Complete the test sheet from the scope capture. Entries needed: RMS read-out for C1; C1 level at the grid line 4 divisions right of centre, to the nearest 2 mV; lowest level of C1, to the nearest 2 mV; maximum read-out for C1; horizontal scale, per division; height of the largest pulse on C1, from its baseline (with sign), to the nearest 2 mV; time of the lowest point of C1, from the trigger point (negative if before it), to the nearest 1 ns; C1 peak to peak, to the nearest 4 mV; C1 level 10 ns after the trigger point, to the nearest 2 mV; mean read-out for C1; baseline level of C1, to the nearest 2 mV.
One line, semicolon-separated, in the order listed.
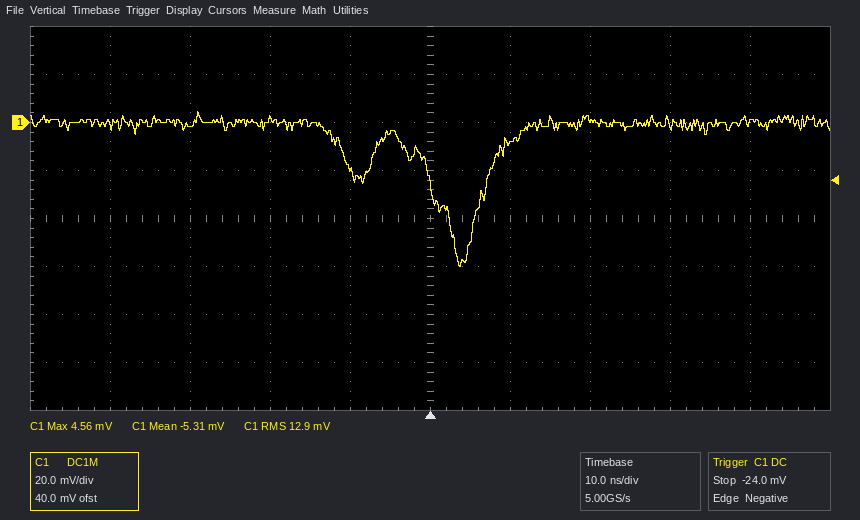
12.9 mV; 0 mV; -60 mV; 4.56 mV; 10 ns; -60 mV; +4 ns; 64 mV; -8 mV; -5.31 mV; 0 mV
